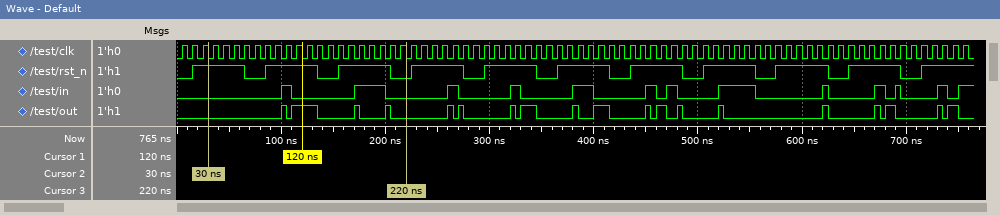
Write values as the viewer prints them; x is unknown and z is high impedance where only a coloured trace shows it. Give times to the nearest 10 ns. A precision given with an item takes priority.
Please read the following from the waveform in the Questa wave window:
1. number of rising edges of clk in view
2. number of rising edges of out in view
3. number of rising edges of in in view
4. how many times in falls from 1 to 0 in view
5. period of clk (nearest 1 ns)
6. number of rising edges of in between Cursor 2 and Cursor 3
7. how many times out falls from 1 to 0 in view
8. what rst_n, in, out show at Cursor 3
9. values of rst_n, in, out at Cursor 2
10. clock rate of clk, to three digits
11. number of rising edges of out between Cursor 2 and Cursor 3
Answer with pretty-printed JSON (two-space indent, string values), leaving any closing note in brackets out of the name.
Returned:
{
  "number of rising edges of clk in view": "76",
  "number of rising edges of out in view": "19",
  "number of rising edges of in in view": "13",
  "how many times in falls from 1 to 0 in view": "12",
  "period of clk": "10 ns",
  "number of rising edges of in between Cursor 2 and Cursor 3": "2",
  "how many times out falls from 1 to 0 in view": "19",
  "what rst_n, in, out show at Cursor 3": "rst_n=0, in=0, out=0",
  "values of rst_n, in, out at Cursor 2": "rst_n=1, in=0, out=0",
  "clock rate of clk, to three digits": "100 MHz",
  "number of rising edges of out between Cursor 2 and Cursor 3": "4"
}
